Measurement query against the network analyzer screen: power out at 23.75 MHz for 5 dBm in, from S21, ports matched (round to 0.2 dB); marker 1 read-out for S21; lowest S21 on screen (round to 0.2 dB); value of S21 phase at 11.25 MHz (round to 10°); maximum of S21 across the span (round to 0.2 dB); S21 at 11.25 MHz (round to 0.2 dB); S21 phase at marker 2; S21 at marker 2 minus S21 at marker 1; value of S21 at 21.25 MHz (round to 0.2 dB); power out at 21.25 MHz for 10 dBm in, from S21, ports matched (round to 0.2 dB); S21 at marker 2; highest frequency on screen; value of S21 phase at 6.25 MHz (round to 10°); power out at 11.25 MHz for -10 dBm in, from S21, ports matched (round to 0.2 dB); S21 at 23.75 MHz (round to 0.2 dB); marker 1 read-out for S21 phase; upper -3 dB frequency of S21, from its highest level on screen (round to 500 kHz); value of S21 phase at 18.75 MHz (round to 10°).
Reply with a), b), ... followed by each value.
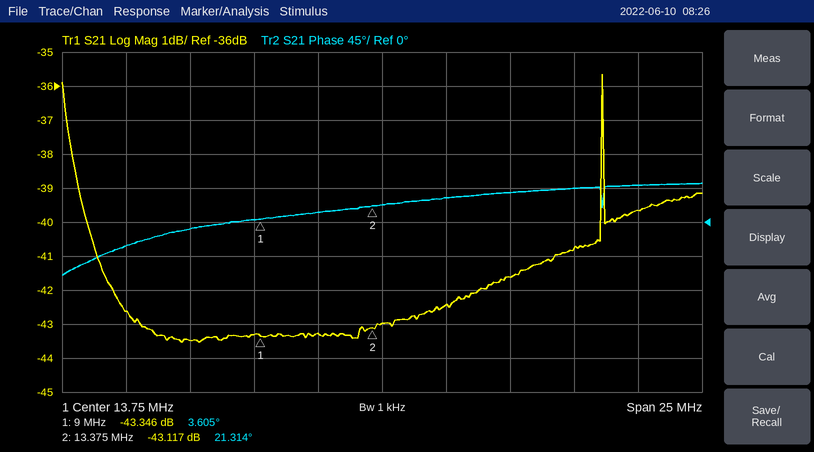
a) -34.6 dBm
b) -43.346 dB
c) -43.6 dB
d) 10°
e) -35.6 dB
f) -43.2 dB
g) 21.314°
h) 0.229 dB
i) -40.8 dB
j) -30.8 dBm
k) -43.117 dB
l) 26.25 MHz
m) -10°
n) -53.2 dBm
o) -39.6 dB
p) 3.605°
q) 22.5 MHz
r) 40°
